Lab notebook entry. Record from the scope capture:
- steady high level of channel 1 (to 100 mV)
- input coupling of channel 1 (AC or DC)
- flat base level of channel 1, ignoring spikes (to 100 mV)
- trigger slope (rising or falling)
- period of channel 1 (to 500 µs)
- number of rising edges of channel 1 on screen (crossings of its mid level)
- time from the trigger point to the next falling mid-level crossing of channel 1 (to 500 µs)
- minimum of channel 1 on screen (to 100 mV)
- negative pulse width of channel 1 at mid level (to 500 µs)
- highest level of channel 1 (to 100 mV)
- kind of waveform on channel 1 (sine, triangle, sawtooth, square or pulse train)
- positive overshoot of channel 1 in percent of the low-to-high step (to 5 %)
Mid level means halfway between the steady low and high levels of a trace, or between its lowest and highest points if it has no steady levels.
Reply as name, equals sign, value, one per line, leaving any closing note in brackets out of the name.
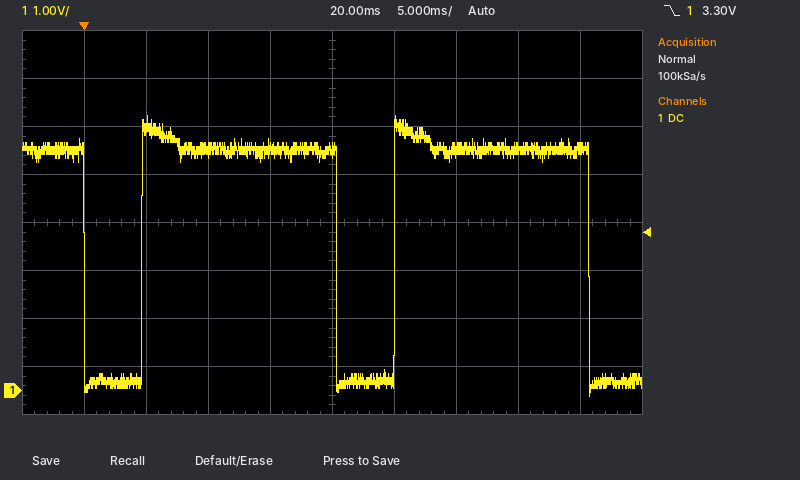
steady high level of channel 1 = 5.0 V
input coupling of channel 1 = DC
flat base level of channel 1, ignoring spikes = 200 mV
trigger slope = falling
period of channel 1 = 20.5 ms
number of rising edges of channel 1 on screen = 2
time from the trigger point to the next falling mid-level crossing of channel 1 = 20.5 ms
minimum of channel 1 on screen = -100 mV
negative pulse width of channel 1 at mid level = 4.5 ms
highest level of channel 1 = 5.7 V
kind of waveform on channel 1 = pulse train
positive overshoot of channel 1 in percent of the low-to-high step = 15 %
